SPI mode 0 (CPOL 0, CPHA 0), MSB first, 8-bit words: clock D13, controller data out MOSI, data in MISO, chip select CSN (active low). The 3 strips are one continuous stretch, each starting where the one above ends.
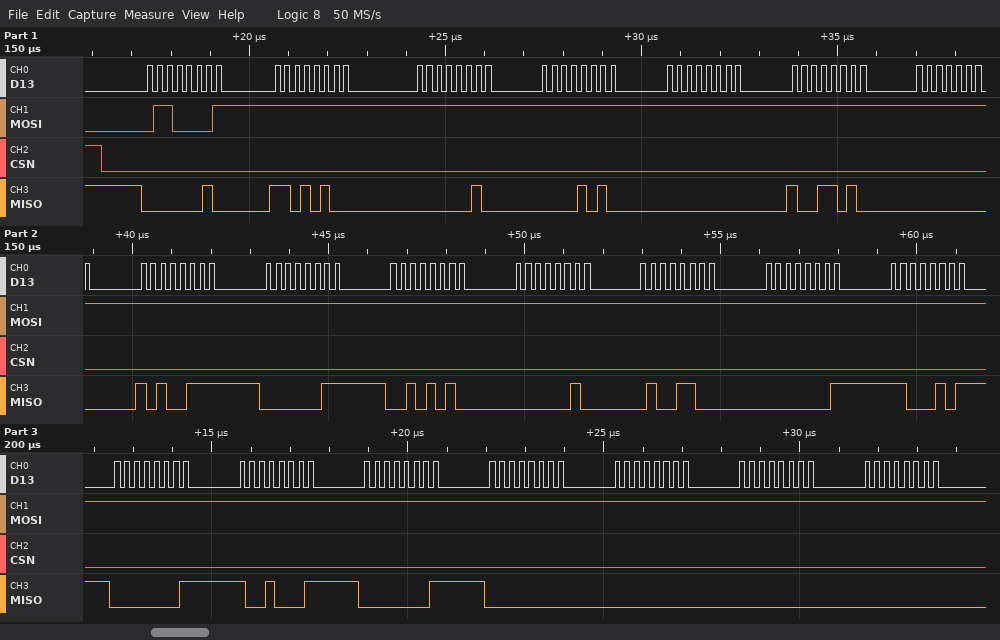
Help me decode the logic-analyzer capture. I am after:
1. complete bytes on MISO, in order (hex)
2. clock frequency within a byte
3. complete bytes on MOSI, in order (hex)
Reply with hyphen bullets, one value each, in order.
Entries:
- 02 D4 02 0A 00 9A 00 A7 03 2A 02 4C 01 C5 01 91 01 00 00 00 00
- 4 MHz
- 61 FF FF FF FF FF FF FF FF FF FF FF FF FF FF FF FF FF FF FF FF
